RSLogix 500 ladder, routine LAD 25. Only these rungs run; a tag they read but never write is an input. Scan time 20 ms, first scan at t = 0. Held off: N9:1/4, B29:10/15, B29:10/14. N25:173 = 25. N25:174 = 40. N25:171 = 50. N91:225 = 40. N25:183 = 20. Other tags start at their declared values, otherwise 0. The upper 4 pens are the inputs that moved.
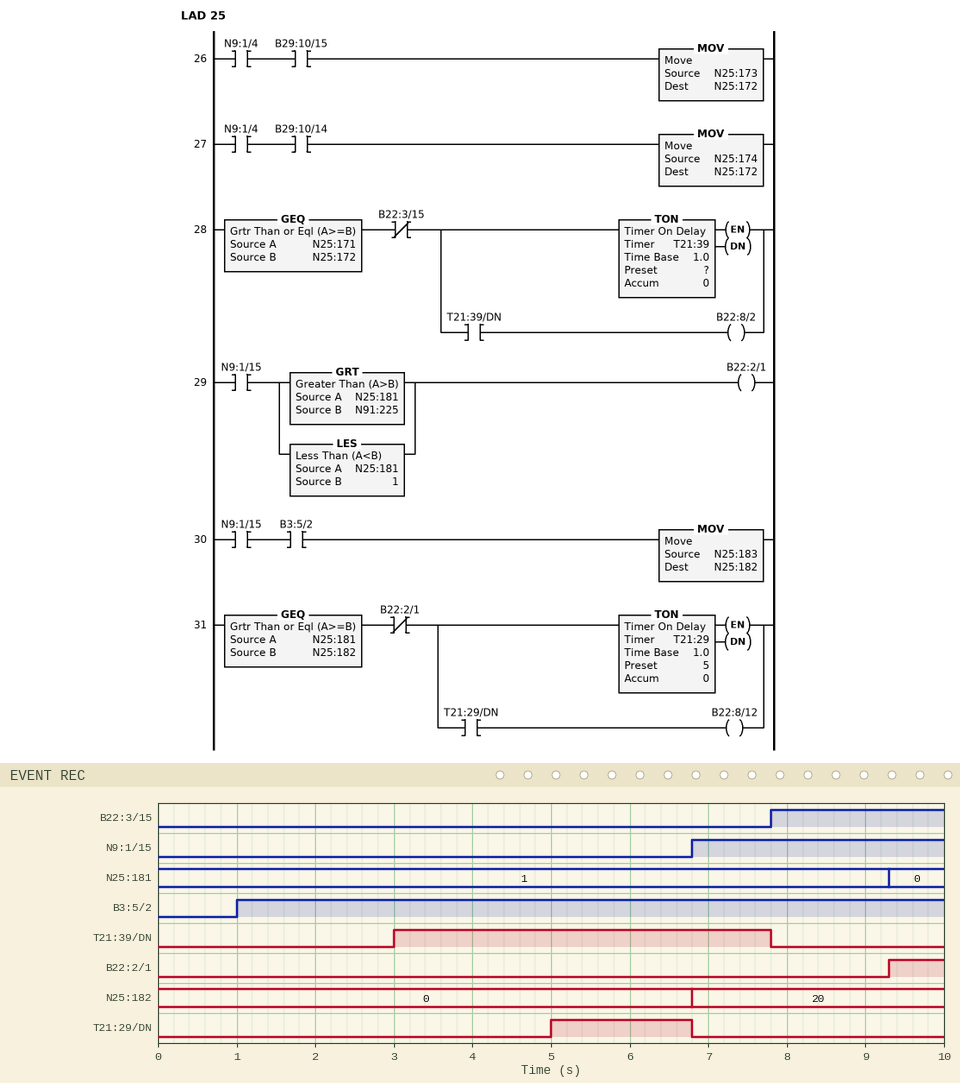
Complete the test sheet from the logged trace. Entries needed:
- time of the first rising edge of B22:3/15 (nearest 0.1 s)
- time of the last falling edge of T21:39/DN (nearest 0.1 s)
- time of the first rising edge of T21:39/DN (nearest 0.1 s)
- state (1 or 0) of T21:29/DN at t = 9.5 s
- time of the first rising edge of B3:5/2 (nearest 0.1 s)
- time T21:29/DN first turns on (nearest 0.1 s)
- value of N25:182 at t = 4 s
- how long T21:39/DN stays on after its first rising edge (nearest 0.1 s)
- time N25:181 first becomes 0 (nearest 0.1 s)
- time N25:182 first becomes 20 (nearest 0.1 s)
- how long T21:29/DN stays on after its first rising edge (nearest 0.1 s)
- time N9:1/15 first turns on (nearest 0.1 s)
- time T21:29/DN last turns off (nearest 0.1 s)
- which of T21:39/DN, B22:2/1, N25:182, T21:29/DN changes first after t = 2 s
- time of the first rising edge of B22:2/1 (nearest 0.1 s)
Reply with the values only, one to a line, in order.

7.8 s
7.8 s
3.0 s
0
1.0 s
5.0 s
0
4.8 s
9.3 s
6.8 s
1.8 s
6.8 s
6.8 s
T21:39/DN
9.3 s
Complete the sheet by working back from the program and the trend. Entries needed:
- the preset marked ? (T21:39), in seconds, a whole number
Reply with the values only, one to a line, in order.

3 s
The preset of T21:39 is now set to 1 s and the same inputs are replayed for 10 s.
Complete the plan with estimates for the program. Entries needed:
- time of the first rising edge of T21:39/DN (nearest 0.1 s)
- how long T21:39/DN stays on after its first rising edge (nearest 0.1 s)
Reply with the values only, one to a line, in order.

1.0 s
6.8 s
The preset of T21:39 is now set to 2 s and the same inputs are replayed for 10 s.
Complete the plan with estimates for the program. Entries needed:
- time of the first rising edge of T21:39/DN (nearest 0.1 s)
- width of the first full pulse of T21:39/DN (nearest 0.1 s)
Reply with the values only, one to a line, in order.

2.0 s
5.8 s
